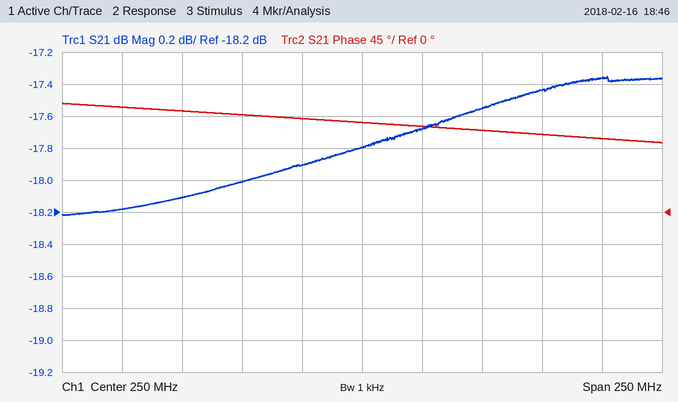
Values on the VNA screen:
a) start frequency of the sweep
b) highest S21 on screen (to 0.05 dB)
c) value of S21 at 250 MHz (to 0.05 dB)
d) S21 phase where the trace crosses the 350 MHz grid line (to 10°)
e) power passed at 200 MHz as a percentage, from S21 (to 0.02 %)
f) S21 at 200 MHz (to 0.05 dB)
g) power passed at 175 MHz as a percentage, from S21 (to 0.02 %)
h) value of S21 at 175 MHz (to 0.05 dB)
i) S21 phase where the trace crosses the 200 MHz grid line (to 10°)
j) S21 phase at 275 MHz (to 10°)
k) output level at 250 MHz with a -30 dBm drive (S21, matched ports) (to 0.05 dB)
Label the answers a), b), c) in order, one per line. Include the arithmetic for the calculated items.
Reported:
a) 125 MHz
b) -17.35 dB
c) -17.80 dB
d) 100°
e) 10^(-18/10) ≈ 1.58 %
f) -18.00 dB
g) 10^(-18.1/10) ≈ 1.55 %, so 1.54 % to the nearest 0.02 %
h) -18.10 dB
i) 140°
j) 120°
k) -30 dBm + (-17.80 dB) = -47.80 dBm
